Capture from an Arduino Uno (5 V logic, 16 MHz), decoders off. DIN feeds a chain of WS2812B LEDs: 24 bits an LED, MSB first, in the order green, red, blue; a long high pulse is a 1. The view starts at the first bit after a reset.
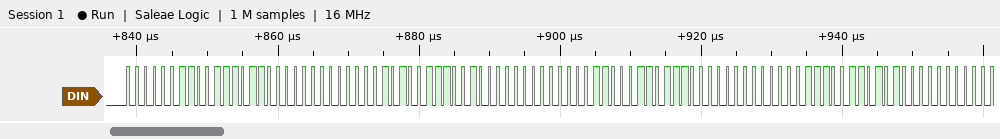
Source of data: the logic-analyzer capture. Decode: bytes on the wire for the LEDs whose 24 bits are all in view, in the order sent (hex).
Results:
03 3B 00 05 39 00 06 37 00 07 35 00
